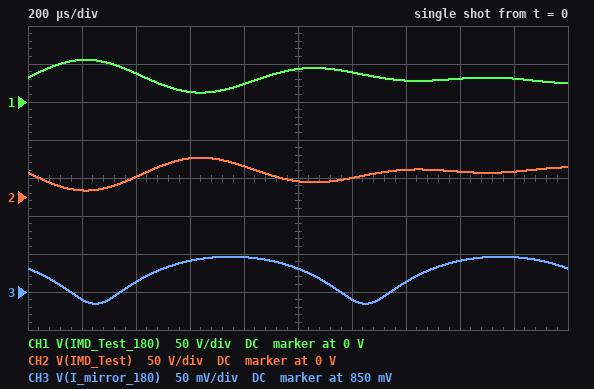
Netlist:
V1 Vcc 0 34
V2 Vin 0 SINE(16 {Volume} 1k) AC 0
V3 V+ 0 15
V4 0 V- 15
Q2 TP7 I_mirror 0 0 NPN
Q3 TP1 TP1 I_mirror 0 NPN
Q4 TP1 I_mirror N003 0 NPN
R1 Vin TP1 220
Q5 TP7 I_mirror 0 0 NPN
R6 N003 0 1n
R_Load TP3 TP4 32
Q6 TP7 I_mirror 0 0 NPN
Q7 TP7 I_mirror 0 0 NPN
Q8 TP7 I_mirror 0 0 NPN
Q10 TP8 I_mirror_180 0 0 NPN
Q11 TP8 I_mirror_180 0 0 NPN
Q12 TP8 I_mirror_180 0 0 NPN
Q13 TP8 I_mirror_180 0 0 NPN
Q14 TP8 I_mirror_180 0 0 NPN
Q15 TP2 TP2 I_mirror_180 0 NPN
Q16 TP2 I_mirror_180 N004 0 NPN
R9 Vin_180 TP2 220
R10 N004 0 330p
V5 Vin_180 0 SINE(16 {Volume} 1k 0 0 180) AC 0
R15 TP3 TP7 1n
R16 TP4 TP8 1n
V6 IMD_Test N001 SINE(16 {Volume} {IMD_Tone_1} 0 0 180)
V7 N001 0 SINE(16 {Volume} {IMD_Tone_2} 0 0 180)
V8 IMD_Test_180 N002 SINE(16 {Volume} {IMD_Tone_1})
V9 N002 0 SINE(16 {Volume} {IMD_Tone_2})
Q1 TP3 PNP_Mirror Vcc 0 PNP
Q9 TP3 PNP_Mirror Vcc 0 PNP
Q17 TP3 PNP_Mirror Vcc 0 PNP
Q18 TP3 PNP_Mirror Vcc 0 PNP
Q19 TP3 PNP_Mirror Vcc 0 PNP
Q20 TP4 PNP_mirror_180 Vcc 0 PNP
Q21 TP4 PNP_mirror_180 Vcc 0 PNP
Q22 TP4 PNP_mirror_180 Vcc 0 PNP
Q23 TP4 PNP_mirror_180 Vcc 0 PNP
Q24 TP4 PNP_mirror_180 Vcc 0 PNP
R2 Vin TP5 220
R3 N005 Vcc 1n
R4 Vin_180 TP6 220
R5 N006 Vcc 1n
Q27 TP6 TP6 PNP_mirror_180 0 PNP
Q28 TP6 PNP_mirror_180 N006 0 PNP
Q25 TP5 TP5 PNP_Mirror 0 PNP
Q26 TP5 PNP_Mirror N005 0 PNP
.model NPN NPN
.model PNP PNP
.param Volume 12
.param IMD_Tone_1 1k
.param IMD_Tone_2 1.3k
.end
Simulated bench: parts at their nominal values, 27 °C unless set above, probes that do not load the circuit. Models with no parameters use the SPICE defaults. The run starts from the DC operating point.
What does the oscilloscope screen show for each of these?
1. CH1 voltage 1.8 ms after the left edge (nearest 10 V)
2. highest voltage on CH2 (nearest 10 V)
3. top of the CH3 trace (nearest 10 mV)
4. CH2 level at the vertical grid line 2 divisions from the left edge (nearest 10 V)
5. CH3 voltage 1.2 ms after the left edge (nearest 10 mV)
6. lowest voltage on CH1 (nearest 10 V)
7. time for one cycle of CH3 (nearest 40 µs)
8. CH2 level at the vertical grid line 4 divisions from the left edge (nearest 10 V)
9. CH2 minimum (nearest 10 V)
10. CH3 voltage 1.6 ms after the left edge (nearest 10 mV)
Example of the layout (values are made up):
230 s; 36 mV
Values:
30 V; 50 V; 900 mV; 30 V; 840 mV; 10 V; 1.00 ms; 40 V; 10 V; 890 mV
